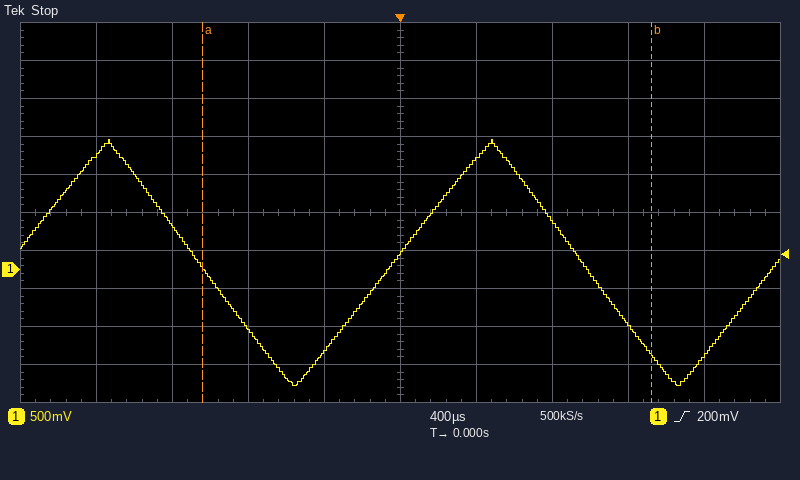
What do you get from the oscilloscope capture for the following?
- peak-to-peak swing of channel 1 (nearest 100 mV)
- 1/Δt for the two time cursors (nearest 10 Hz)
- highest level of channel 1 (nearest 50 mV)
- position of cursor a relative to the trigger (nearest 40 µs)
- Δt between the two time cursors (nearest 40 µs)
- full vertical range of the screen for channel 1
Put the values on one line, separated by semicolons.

3.20 V; 420 Hz; 1.70 V; -1.04 ms; 2.36 ms; 5 V
